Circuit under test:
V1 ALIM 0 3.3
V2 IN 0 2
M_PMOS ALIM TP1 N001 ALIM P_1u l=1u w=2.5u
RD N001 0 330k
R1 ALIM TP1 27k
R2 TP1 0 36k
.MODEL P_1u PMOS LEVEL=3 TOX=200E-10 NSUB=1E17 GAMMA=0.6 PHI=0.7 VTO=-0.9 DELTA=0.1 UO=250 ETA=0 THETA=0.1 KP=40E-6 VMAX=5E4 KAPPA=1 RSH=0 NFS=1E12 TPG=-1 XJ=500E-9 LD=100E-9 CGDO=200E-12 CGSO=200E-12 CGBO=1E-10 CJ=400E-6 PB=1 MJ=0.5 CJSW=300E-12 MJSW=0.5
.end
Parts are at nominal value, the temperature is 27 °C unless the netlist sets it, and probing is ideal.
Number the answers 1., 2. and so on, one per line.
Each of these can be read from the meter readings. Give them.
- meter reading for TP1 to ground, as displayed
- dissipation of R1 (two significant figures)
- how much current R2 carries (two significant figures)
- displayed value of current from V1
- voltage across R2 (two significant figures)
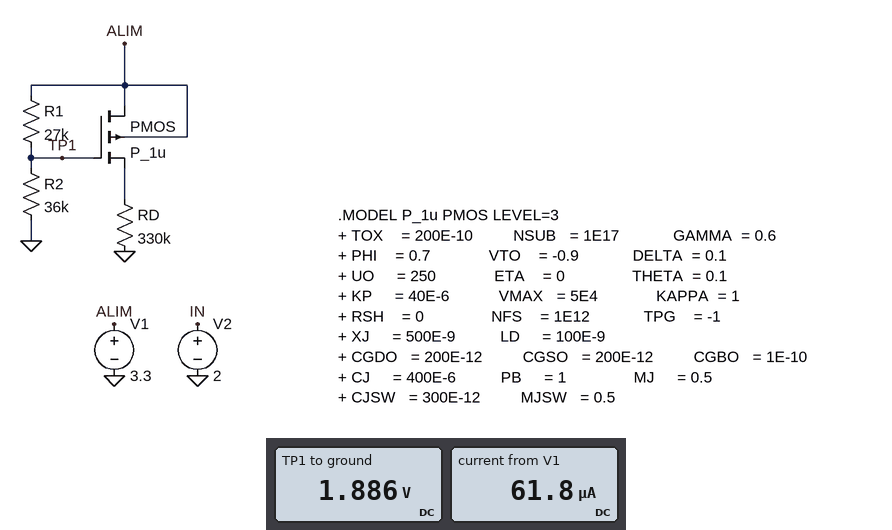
1. 1.886 V
2. 74 µW
3. 52 µA
4. 61.8 µA
5. 1.9 V
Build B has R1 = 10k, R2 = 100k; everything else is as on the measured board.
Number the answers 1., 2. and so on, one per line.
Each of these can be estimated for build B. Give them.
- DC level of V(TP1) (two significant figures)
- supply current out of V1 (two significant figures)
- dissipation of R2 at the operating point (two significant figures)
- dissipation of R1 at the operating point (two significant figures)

1. 3.0 V
2. 30 µA
3. 90 µW
4. 9.0 µW
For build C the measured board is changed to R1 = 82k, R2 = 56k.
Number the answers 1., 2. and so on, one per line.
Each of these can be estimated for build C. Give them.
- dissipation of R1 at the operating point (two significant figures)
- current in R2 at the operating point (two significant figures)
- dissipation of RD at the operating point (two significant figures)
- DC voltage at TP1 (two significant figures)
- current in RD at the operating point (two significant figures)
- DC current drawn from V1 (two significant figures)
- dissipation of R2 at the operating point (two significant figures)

1. 47 µW
2. 24 µA
3. 31 µW
4. 1.3 V
5. 9.7 µA
6. 34 µA
7. 32 µW
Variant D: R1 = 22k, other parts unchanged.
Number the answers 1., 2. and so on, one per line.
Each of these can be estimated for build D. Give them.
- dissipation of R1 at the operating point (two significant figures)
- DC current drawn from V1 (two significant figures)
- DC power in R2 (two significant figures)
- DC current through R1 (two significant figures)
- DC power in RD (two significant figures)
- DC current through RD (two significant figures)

1. 71 µW
2. 65 µA
3. 120 µW
4. 57 µA
5. 19 µW
6. 7.7 µA
